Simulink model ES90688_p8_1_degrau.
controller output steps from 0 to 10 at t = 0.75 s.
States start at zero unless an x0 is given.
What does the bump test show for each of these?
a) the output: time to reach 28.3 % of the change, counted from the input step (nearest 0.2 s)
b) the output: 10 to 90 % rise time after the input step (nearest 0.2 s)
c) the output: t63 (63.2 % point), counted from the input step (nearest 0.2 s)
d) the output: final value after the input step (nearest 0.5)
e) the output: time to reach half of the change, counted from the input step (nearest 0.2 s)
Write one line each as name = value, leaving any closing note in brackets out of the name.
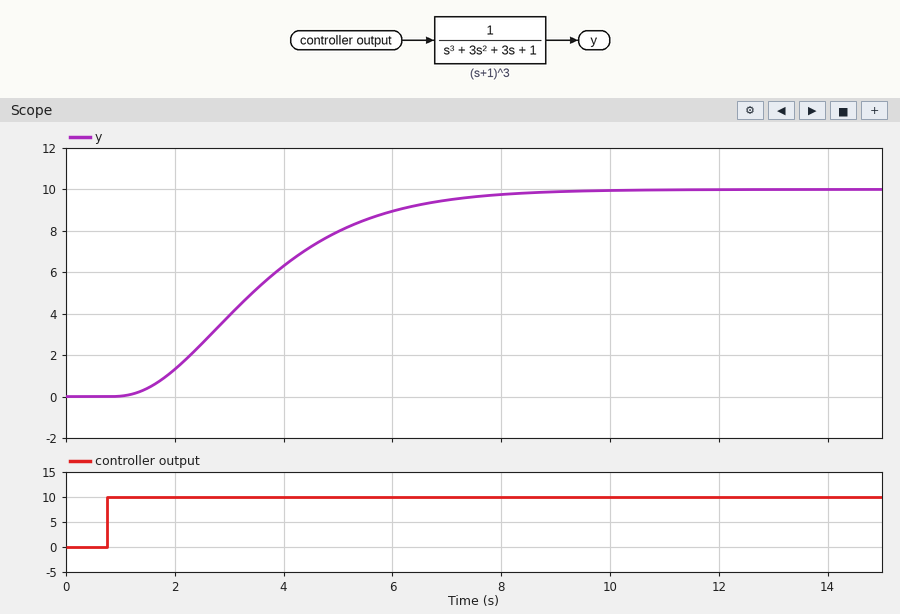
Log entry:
the output: time to reach 28.3 % of the change, counted from the input step = 1.8 s
the output: 10 to 90 % rise time after the input step = 4.2 s
the output: t63 (63.2 % point), counted from the input step = 3.2 s
the output: final value after the input step = 10.0
the output: time to reach half of the change, counted from the input step = 2.6 s
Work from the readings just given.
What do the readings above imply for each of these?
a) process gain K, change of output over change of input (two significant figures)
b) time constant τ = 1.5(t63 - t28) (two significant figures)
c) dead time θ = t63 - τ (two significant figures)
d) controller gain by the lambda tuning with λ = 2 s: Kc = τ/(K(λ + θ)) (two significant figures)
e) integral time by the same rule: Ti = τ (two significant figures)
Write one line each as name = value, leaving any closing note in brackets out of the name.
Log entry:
process gain K, change of output over change of input = 1.0
time constant τ = 1.5(t63 - t28) = 2.1 s
dead time θ = t63 - τ = 1.1 s
controller gain by the lambda tuning with λ = 2 s: Kc = τ/(K(λ + θ)) = 0.68
integral time by the same rule: Ti = τ = 2.1 s
